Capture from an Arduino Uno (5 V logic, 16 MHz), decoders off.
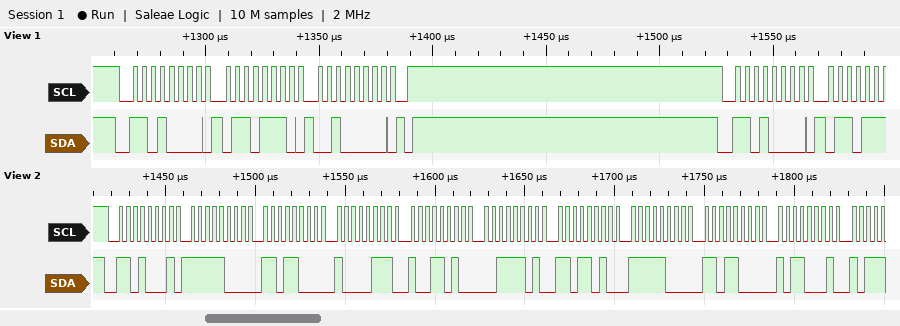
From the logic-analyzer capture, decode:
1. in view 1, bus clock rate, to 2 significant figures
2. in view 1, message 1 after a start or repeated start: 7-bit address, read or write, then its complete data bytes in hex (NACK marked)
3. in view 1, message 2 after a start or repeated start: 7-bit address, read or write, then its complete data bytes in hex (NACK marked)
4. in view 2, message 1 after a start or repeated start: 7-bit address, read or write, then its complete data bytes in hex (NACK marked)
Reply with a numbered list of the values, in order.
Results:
1. 250 kHz
2. 0x68 write: 6E 20
3. 0x68 write
4. 0x68 read: F8 D8 87 9A 3D DA F8 D8 B1
